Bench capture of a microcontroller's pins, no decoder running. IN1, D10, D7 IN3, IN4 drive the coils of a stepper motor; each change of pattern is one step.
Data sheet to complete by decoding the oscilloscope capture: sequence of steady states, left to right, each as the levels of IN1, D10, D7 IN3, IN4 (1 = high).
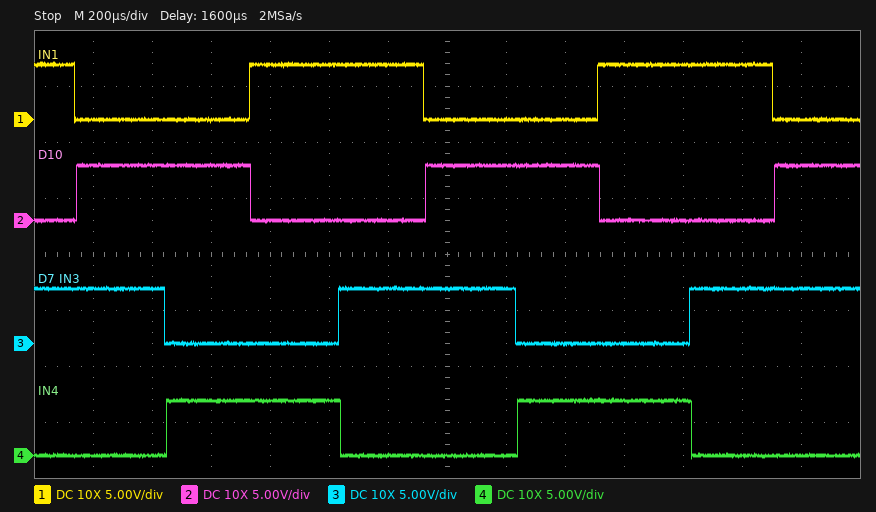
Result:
1010 0110 0101 1001 1010 0110 0101 1001 1010 0110
